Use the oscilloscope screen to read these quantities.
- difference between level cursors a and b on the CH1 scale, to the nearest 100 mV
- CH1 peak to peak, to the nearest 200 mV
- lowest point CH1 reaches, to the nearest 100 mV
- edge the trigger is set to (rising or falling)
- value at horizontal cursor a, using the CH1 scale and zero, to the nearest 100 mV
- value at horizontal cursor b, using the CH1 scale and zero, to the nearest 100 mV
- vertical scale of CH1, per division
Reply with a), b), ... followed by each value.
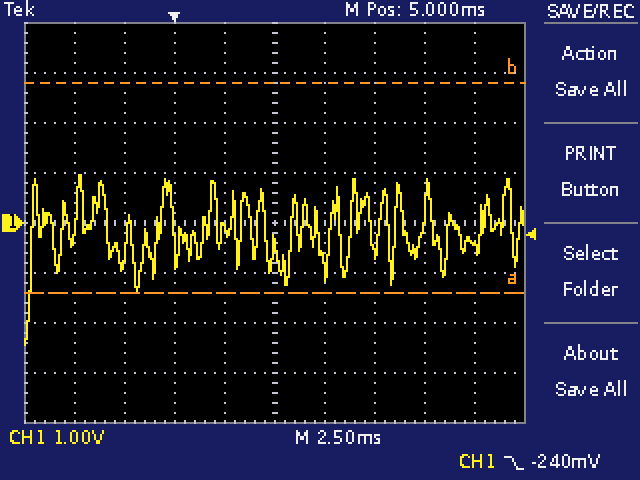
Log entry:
a) 4.2 V
b) 3.4 V
c) -2.4 V
d) falling
e) -1.4 V
f) 2.8 V
g) 1 V
